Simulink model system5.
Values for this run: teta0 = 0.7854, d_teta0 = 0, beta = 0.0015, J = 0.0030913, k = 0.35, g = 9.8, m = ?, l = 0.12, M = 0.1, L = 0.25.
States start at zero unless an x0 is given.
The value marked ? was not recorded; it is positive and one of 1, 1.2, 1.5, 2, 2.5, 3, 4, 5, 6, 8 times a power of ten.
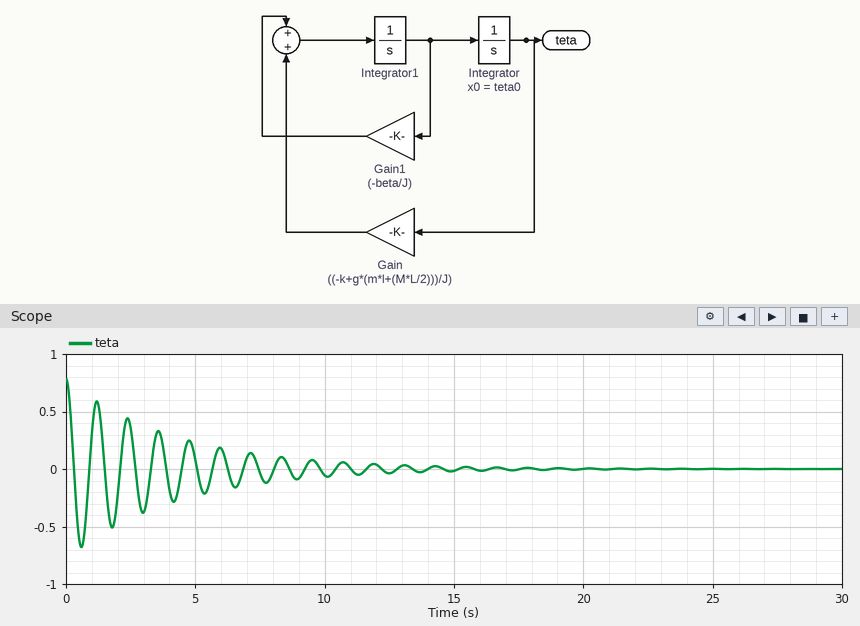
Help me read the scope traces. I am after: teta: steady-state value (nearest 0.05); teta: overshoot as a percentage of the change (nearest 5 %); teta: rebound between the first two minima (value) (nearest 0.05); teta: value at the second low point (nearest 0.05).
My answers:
0.00
85 %
0.60
-0.50
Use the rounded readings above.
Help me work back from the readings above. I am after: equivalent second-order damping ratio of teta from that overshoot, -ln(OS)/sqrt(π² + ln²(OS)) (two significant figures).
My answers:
0.052
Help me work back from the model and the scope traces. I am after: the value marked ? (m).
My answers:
0.12
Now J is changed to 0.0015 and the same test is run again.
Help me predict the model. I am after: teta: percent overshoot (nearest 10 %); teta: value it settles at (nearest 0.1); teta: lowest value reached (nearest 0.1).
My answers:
80 %
0.0
-0.6
